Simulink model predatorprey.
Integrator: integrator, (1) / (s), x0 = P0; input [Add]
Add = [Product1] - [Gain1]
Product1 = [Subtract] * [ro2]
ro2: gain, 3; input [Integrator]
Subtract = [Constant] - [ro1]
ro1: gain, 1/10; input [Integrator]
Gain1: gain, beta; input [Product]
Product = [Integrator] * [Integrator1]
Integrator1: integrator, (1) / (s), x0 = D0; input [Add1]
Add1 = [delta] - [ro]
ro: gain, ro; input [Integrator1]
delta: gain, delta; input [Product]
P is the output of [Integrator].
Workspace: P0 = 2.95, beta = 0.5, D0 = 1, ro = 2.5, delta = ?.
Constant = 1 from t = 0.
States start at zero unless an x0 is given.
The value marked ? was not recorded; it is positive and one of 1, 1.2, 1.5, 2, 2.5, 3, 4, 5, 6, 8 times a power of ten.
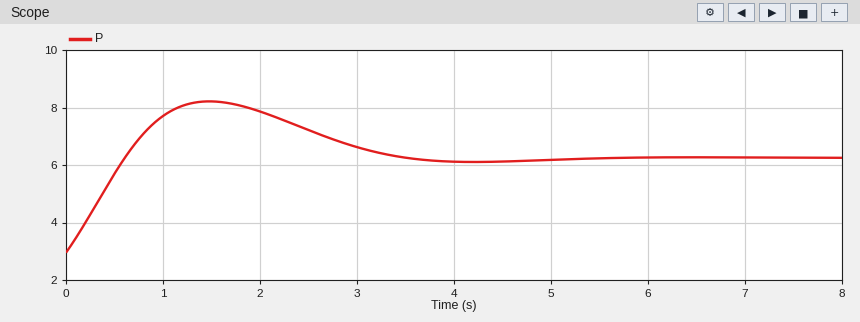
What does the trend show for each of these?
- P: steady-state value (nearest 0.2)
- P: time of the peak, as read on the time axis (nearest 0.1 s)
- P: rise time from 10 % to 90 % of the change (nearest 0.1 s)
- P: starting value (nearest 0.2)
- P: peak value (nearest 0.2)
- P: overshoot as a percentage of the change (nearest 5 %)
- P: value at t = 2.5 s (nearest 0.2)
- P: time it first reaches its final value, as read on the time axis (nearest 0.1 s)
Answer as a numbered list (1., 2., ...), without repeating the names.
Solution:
1. 6.2
2. 1.5 s
3. 0.5 s
4. 3.0
5. 8.2
6. 60 %
7. 7.2
8. 0.6 s
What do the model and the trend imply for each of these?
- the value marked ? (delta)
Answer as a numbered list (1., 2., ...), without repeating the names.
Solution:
1. 0.4
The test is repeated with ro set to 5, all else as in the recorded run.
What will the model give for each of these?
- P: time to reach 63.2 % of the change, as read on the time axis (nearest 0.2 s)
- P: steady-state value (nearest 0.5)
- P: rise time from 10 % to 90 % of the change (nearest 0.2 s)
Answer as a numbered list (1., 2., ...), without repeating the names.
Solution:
1. 0.8 s
2. 10.0
3. 1.2 s
